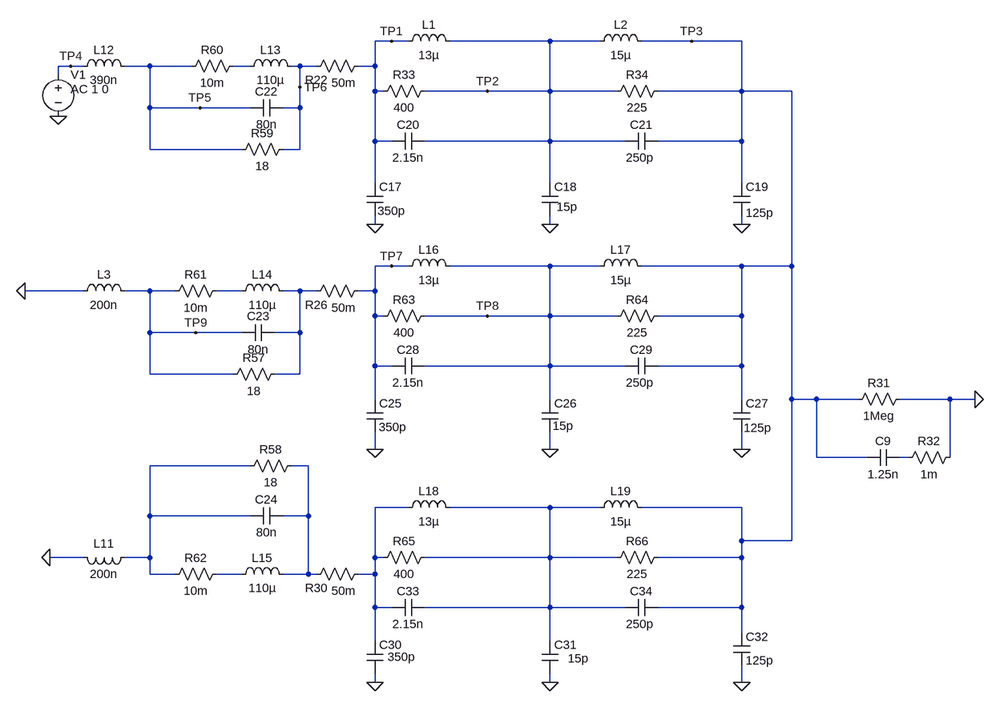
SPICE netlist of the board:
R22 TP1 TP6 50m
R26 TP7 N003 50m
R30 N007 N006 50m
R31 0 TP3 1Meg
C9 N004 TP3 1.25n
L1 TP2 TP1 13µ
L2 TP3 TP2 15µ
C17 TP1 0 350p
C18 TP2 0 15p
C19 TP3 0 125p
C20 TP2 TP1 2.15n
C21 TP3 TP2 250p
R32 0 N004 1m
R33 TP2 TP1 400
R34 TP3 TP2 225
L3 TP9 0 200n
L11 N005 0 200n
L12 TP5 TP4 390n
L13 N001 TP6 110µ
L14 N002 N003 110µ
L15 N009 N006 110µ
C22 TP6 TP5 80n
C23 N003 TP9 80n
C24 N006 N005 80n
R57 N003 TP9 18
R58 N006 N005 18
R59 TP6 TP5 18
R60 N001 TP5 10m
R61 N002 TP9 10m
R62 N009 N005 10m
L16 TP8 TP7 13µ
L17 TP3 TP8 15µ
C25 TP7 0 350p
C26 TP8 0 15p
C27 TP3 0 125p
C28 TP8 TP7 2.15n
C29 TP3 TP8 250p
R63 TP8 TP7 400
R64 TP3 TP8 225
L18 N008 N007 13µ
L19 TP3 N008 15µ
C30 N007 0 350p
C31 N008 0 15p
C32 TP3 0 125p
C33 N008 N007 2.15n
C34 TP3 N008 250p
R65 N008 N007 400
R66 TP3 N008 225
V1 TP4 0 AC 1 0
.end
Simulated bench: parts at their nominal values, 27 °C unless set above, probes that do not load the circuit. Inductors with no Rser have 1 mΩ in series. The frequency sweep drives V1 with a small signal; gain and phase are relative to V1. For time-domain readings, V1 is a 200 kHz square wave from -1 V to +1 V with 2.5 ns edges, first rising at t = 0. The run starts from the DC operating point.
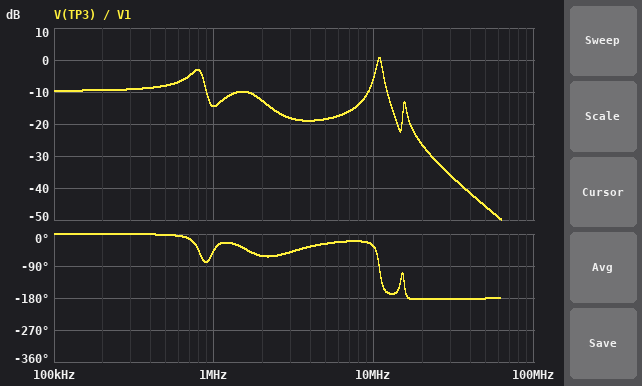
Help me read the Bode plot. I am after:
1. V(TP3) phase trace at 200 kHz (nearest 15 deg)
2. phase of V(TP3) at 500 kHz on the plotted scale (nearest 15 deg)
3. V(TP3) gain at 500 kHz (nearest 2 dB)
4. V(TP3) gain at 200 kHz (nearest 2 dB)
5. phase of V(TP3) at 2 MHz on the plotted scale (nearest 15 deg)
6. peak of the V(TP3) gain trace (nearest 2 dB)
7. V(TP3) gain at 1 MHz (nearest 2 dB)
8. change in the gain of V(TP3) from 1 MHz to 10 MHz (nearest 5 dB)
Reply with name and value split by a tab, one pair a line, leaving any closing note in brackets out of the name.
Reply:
V(TP3) phase trace at 200 kHz	0 deg
phase of V(TP3) at 500 kHz on the plotted scale	0 deg
V(TP3) gain at 500 kHz	-8 dB
V(TP3) gain at 200 kHz	-10 dB
phase of V(TP3) at 2 MHz on the plotted scale	-60 deg
peak of the V(TP3) gain trace	0 dB
V(TP3) gain at 1 MHz	-14 dB
change in the gain of V(TP3) from 1 MHz to 10 MHz	10 dB
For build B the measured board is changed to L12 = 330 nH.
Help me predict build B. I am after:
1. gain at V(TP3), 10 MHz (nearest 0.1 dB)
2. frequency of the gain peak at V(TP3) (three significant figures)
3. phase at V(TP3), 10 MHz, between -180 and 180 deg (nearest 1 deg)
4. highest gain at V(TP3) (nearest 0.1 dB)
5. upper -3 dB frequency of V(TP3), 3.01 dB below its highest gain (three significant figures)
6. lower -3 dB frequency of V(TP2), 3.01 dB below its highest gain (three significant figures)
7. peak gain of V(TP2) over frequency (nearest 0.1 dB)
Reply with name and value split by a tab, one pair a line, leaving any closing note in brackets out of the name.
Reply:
gain at V(TP3), 10 MHz	-10.0 dB
frequency of the gain peak at V(TP3)	11.7 MHz
phase at V(TP3), 10 MHz, between -180 and 180 deg	-22 deg
highest gain at V(TP3)	1.0 dB
upper -3 dB frequency of V(TP3), 3.01 dB below its highest gain	12.2 MHz
lower -3 dB frequency of V(TP2), 3.01 dB below its highest gain	11.3 MHz
peak gain of V(TP2) over frequency	21.3 dB
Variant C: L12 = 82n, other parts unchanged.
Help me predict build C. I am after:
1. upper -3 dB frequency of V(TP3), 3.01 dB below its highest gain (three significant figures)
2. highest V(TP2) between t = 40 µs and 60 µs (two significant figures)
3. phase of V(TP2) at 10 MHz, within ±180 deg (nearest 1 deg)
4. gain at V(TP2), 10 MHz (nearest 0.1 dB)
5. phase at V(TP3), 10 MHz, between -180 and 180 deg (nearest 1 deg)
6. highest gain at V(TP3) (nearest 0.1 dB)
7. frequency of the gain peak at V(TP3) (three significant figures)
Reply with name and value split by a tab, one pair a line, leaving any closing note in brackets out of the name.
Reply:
upper -3 dB frequency of V(TP3), 3.01 dB below its highest gain	24.0 MHz
highest V(TP2) between t = 40 µs and 60 µs	2.9 V
phase of V(TP2) at 10 MHz, within ±180 deg	0 deg
gain at V(TP2), 10 MHz	0.8 dB
phase at V(TP3), 10 MHz, between -180 and 180 deg	-10 deg
highest gain at V(TP3)	9.1 dB
frequency of the gain peak at V(TP3)	23.6 MHz
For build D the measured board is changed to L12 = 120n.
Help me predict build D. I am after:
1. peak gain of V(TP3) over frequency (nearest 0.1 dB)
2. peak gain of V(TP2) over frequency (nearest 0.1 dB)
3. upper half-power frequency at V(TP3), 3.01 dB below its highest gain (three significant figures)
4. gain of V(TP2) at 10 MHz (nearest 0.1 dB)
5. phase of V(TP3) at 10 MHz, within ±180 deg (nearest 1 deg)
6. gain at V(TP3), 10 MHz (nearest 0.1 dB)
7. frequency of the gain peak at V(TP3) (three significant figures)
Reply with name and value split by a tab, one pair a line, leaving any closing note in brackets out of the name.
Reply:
peak gain of V(TP3) over frequency	8.4 dB
peak gain of V(TP2) over frequency	26.2 dB
upper half-power frequency at V(TP3), 3.01 dB below its highest gain	19.9 MHz
gain of V(TP2) at 10 MHz	1.7 dB
phase of V(TP3) at 10 MHz, within ±180 deg	-11 deg
gain at V(TP3), 10 MHz	-18.2 dB
frequency of the gain peak at V(TP3)	19.5 MHz
